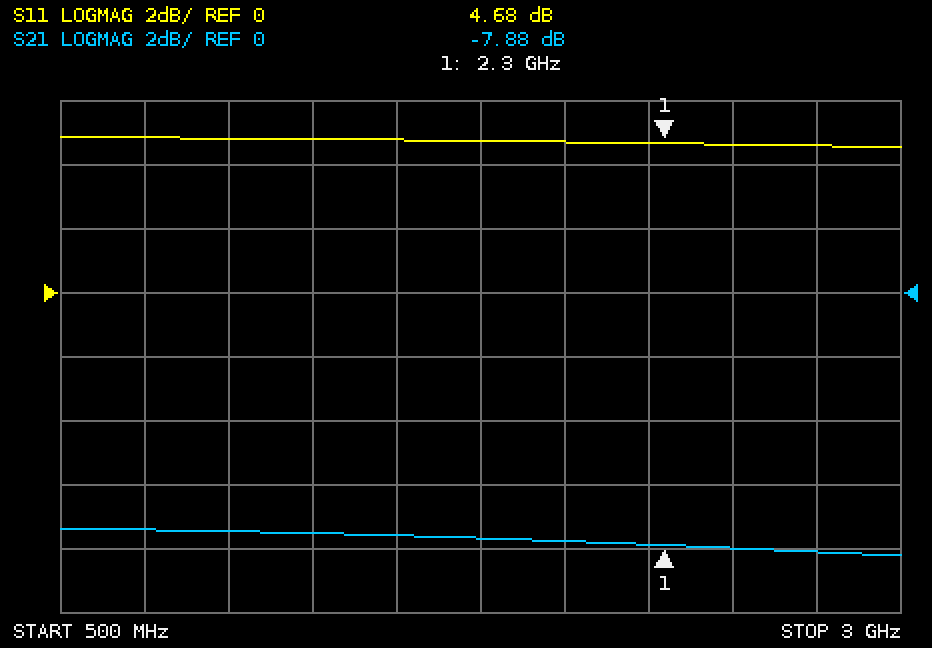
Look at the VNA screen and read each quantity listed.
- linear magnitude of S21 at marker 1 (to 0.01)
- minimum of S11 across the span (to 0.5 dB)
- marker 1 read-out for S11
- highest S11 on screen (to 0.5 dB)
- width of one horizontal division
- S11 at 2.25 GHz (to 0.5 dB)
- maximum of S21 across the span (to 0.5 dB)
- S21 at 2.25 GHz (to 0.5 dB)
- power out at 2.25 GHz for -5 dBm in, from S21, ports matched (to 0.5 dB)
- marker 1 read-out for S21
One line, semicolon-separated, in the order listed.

0.40; 4.5 dB; 4.68 dB; 5.0 dB; 250 MHz; 4.5 dB; -7.5 dB; -8.0 dB; -13.0 dBm; -7.88 dB
